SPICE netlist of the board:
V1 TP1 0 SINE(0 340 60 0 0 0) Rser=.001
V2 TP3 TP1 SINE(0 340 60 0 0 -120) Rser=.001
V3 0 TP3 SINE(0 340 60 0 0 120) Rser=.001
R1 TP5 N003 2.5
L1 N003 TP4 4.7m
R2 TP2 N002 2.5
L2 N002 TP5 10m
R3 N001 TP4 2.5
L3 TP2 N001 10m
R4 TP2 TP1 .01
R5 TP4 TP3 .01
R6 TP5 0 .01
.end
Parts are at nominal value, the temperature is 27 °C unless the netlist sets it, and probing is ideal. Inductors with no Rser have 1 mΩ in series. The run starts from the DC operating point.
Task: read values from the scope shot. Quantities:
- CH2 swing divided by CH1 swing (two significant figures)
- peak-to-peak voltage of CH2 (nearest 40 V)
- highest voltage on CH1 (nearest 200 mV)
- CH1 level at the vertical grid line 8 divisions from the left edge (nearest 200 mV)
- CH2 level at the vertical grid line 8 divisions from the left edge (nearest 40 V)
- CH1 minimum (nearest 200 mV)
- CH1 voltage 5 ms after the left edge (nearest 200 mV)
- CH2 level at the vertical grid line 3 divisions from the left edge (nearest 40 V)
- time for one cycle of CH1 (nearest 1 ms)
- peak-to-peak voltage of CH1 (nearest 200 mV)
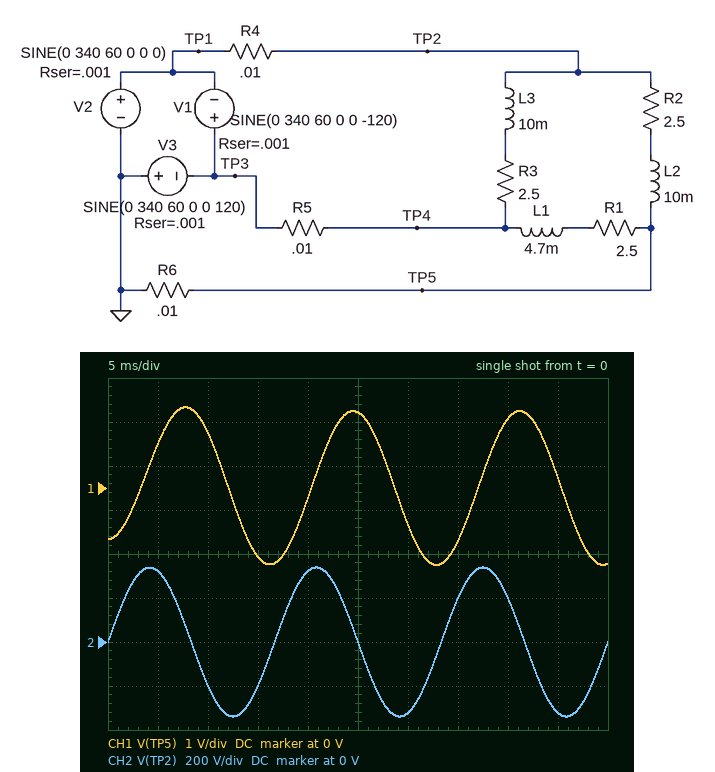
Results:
190
680 V
1.8 V
1.6 V
200 V
-1.8 V
1.0 V
-200 V
17 ms
3.6 V
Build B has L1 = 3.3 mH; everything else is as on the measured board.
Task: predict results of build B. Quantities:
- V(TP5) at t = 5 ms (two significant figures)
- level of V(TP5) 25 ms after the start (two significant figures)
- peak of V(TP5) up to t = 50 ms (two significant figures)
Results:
1.2 V
1.8 V
2.0 V
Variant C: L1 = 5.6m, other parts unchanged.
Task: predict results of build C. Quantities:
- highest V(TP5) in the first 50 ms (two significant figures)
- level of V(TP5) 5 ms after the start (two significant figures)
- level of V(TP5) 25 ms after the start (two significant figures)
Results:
1.7 V
900 mV
1.6 V
